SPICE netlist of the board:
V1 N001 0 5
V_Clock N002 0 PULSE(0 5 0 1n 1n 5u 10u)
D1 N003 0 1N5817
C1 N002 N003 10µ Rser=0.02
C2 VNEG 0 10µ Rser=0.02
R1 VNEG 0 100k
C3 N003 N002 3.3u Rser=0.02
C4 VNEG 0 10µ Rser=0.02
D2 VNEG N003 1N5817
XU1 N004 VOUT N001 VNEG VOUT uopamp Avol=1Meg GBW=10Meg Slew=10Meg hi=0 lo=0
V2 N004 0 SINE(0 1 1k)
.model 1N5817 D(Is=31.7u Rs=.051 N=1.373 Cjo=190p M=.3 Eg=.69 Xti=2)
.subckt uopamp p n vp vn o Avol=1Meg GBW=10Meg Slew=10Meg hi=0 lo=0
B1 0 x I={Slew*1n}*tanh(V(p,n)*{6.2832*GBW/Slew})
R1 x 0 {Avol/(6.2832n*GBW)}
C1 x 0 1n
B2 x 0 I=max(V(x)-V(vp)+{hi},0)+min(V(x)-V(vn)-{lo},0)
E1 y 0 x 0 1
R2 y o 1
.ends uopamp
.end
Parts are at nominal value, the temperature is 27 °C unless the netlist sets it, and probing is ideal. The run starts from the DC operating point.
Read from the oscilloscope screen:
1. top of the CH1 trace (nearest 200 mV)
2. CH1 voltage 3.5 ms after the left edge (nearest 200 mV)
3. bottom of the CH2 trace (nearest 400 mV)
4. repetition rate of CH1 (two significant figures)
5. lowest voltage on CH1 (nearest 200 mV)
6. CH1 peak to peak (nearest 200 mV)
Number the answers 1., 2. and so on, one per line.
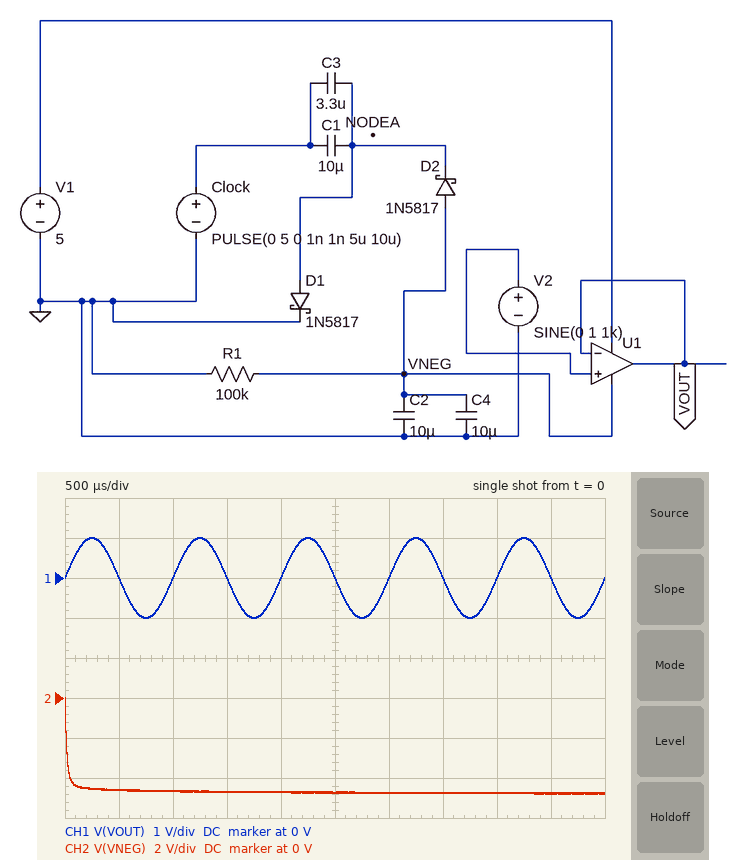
1. 1.0 V
2. 0 V
3. -4.8 V
4. 1.0 kHz
5. -1.0 V
6. 2.0 V
